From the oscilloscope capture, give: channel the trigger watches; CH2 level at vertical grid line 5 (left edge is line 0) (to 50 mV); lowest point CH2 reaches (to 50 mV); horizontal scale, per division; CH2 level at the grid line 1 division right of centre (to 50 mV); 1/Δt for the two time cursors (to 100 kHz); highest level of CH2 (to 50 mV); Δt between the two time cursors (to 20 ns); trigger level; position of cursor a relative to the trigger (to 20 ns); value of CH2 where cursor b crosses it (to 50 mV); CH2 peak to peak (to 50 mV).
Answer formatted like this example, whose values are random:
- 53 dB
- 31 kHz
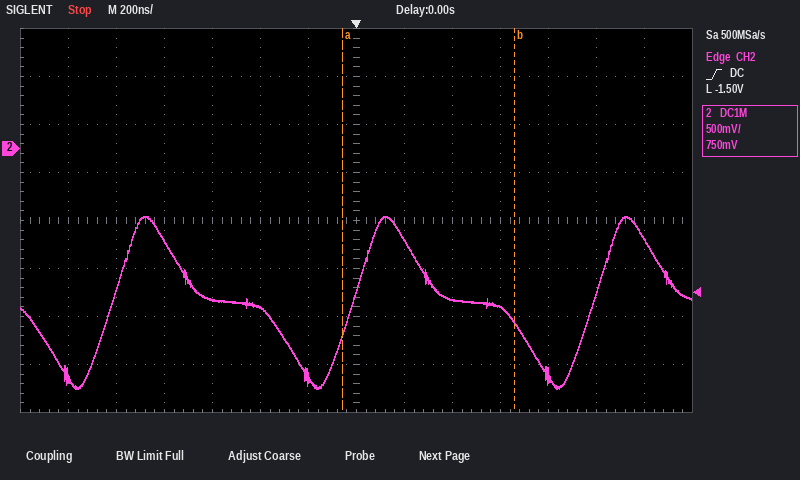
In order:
- CH2
- -1.65 V
- -2.50 V
- 200 ns
- -950 mV
- 1.4 MHz
- -700 mV
- 720 ns
- -1.50 V
- -60 ns
- -1.80 V
- 1.80 V
